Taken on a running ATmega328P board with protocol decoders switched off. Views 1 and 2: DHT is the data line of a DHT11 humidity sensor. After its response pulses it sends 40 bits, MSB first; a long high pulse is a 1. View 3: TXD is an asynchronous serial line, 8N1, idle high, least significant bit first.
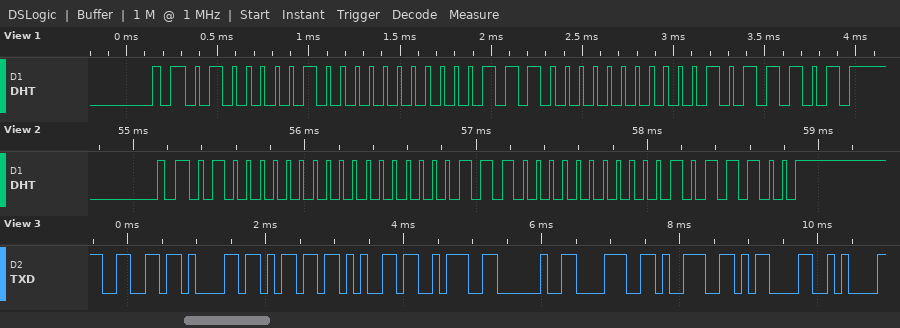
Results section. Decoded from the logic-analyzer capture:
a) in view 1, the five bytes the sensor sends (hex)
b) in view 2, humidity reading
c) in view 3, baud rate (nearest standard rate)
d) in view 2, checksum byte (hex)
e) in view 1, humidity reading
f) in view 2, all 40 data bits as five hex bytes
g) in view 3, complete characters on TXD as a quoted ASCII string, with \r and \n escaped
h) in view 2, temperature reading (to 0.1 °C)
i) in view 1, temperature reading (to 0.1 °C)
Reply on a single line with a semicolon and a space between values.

41 00 1C 00 5D; 64 %; 9600 baud; 0x5C; 65 %; 40 00 1C 00 5C; "fame: 89\r\n"; 28.0 °C; 28.0 °C
